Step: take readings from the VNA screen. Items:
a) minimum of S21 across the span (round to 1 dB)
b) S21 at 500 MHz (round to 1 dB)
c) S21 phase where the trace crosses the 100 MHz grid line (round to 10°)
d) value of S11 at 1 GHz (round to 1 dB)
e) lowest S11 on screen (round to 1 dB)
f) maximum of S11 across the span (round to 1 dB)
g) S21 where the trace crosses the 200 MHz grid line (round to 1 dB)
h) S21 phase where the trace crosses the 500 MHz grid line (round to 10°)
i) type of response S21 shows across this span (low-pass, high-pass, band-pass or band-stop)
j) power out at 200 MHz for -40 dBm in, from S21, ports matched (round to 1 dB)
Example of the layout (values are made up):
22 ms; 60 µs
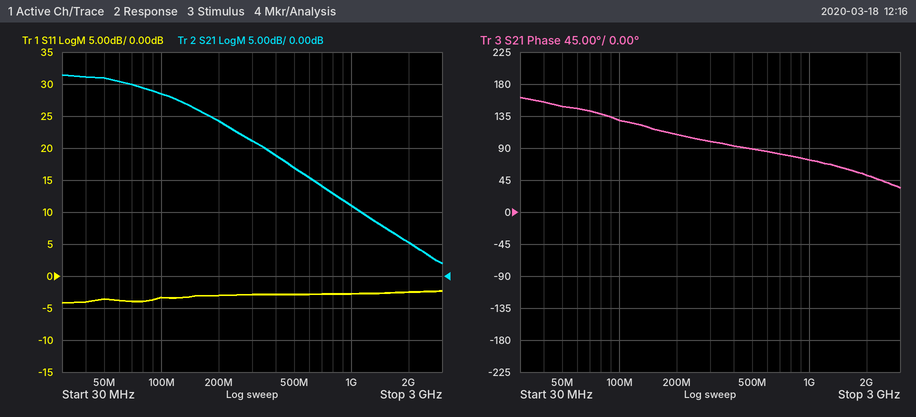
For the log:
2 dB; 17 dB; 130°; -3 dB; -4 dB; -2 dB; 24 dB; 90°; low-pass; -16 dBm
